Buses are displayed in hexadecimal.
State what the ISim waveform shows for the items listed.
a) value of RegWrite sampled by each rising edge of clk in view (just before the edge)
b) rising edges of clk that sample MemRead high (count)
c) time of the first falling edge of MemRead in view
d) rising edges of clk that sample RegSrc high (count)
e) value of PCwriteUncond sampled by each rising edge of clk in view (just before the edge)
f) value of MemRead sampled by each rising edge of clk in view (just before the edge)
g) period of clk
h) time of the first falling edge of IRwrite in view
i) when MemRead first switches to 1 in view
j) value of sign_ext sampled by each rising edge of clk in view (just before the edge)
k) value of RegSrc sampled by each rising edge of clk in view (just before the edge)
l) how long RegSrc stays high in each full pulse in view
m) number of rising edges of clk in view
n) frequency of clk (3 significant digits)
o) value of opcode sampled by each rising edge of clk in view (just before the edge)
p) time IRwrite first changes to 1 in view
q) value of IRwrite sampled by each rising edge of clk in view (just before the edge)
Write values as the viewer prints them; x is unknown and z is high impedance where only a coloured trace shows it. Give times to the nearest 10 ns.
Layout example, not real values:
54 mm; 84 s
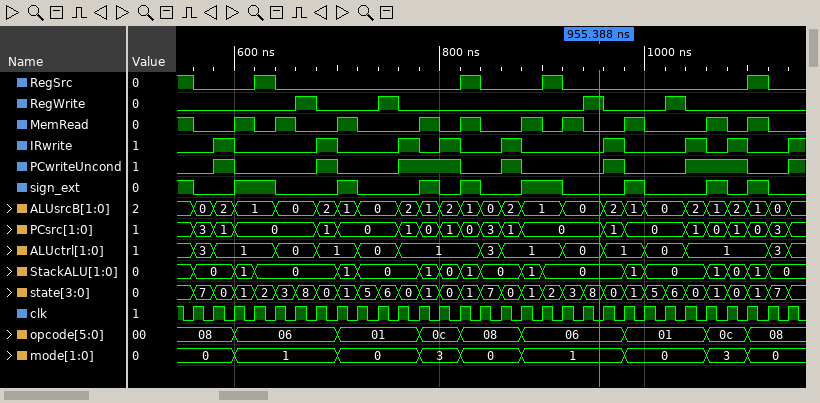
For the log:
0 0 0 0 0 0 1 0 0 0 1 0 0 0 0 0 0 0 0 0 1 0 0 0 1 0 0 0 0 0; 11; 560 ns; 5; 0 0 1 0 0 0 0 1 0 0 0 1 1 1 0 0 1 0 0 0 0 1 0 0 0 1 1 1 0 0; 1 0 0 1 0 1 0 0 1 0 0 0 1 0 1 0 0 1 0 1 0 0 1 0 0 0 1 0 1 0; 20 ns; 600 ns; 600 ns; 1 0 0 1 1 0 0 0 1 0 0 0 1 0 1 0 0 1 1 0 0 0 1 0 0 0 1 0 1 0; 1 0 0 0 1 0 0 0 0 0 0 0 0 0 1 0 0 0 1 0 0 0 0 0 0 0 0 0 1 0; 20 ns, 20 ns, 20 ns, 20 ns; 30; 50.0 MHz; 08, 08, 08, 06, 06, 06, 06, 06, 01, 01, 01, 01, 0c, 0c, 08, 08, 08, 06, 06, 06, 06, 06, 01, 01, 01, 01, 0c, 0c, 08, 08; 580 ns; 0 0 1 0 0 0 0 1 0 0 0 1 0 1 0 0 1 0 0 0 0 1 0 0 0 1 0 1 0 0
